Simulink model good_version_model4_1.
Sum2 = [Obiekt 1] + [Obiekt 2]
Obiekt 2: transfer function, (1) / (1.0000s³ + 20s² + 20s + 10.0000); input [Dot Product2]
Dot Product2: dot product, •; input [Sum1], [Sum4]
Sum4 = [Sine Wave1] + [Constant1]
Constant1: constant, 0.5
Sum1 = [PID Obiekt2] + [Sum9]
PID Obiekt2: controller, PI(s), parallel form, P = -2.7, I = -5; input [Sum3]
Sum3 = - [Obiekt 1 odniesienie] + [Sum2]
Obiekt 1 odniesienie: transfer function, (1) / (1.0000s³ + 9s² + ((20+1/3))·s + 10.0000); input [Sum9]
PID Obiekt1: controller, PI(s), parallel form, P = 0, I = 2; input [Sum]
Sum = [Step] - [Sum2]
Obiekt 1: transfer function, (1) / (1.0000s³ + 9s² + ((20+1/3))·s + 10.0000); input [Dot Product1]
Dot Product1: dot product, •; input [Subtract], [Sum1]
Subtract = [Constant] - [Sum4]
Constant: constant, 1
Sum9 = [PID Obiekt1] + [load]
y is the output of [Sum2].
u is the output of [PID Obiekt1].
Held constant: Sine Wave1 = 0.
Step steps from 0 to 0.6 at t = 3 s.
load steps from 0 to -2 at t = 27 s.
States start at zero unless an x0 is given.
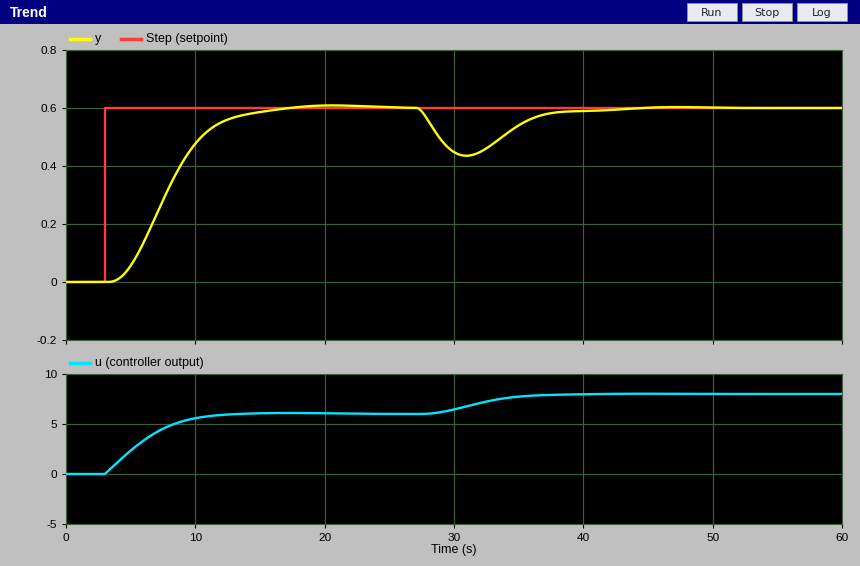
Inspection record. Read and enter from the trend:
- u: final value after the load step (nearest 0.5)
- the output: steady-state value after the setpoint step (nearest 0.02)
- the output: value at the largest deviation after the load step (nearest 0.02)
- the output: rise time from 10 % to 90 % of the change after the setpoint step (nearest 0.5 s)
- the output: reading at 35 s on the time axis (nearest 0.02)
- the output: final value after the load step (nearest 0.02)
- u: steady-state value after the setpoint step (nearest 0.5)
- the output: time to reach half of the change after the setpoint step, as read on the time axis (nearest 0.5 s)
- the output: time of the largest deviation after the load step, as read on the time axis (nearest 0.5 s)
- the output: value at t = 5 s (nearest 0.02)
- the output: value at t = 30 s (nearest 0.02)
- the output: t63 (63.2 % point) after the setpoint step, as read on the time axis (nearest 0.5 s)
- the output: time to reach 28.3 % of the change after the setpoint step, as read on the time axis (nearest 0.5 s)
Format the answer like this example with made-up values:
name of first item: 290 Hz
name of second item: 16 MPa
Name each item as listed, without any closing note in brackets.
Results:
u: final value after the load step: 8.0
the output: steady-state value after the setpoint step: 0.60
the output: value at the largest deviation after the load step: 0.44
the output: rise time from 10 % to 90 % of the change after the setpoint step: 6.5 s
the output: reading at 35 s on the time axis: 0.54
the output: final value after the load step: 0.60
u: steady-state value after the setpoint step: 6.0
the output: time to reach half of the change after the setpoint step, as read on the time axis: 7.5 s
the output: time of the largest deviation after the load step, as read on the time axis: 31.0 s
the output: value at t = 5 s: 0.06
the output: value at t = 30 s: 0.44
the output: t63 (63.2 % point) after the setpoint step, as read on the time axis: 8.5 s
the output: time to reach 28.3 % of the change after the setpoint step, as read on the time axis: 6.5 s
